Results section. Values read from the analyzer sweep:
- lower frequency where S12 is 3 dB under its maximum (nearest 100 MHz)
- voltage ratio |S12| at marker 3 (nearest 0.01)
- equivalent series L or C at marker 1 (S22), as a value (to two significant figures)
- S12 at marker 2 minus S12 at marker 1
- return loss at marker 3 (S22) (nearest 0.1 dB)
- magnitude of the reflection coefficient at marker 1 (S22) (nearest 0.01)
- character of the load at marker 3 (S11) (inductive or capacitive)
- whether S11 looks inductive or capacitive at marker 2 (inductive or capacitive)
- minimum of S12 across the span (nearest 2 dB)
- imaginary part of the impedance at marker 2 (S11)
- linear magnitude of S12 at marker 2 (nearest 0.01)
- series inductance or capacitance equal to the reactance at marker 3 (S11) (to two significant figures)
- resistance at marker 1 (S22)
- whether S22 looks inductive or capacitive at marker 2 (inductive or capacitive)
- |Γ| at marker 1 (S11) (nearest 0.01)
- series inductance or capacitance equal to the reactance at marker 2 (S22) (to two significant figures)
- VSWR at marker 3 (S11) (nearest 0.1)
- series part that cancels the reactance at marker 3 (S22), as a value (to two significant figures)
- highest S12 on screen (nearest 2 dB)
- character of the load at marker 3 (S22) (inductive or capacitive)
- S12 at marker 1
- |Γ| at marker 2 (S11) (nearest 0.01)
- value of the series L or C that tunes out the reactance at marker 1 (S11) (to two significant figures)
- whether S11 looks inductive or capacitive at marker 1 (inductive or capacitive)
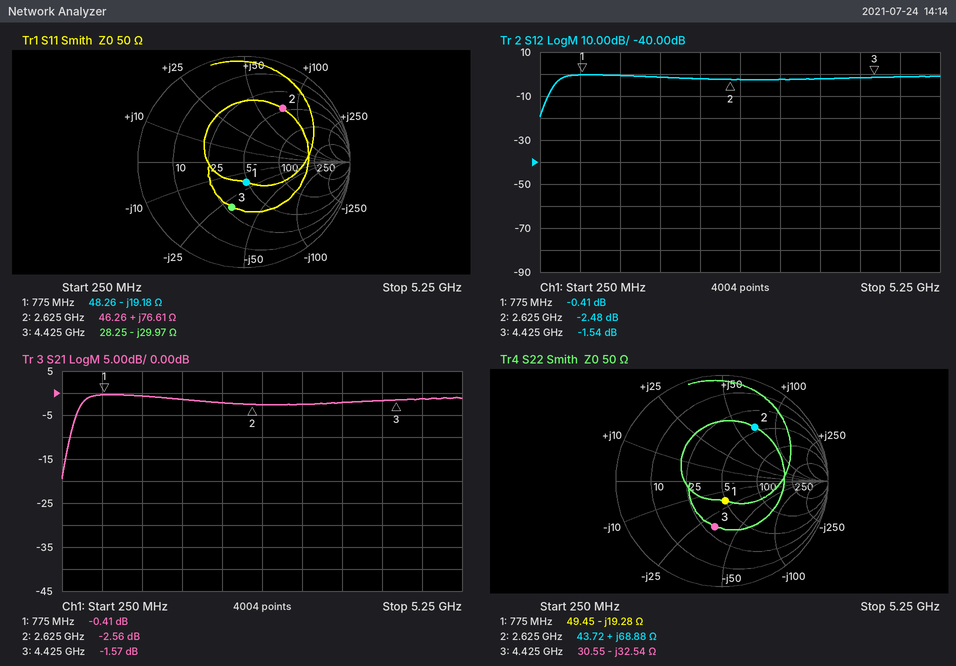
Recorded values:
500 MHz
0.84
11 pF
-2.07 dB
7.2 dB
0.19
capacitive
inductive
-20 dB
+76.61 Ω
0.75
1.2 pF
49.45 Ω
inductive
0.19
4.2 nH
2.6
1.2 nH
0 dB
capacitive
-0.41 dB
0.62
3.9 nH
capacitive
